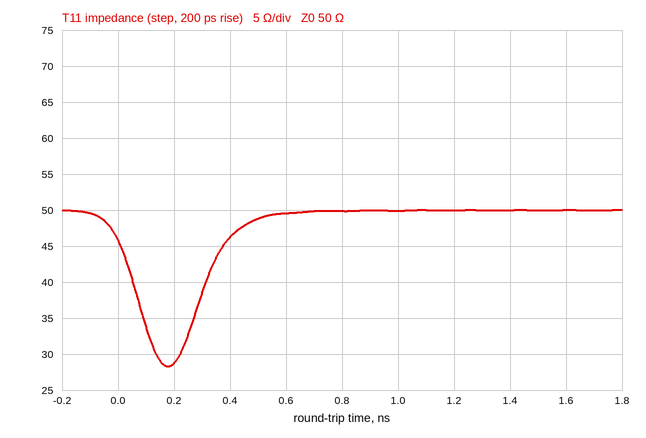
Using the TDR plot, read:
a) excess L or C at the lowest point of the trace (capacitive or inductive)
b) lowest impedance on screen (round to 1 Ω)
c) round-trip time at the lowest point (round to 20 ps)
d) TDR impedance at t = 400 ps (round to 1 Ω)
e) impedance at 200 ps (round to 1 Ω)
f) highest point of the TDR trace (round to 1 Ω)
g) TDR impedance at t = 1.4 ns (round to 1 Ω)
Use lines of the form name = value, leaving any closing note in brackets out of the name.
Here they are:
excess L or C at the lowest point of the trace = capacitive
lowest impedance on screen = 28 Ω
round-trip time at the lowest point = 180 ps
TDR impedance at t = 400 ps = 46 Ω
impedance at 200 ps = 29 Ω
highest point of the TDR trace = 50 Ω
TDR impedance at t = 1.4 ns = 50 Ω
